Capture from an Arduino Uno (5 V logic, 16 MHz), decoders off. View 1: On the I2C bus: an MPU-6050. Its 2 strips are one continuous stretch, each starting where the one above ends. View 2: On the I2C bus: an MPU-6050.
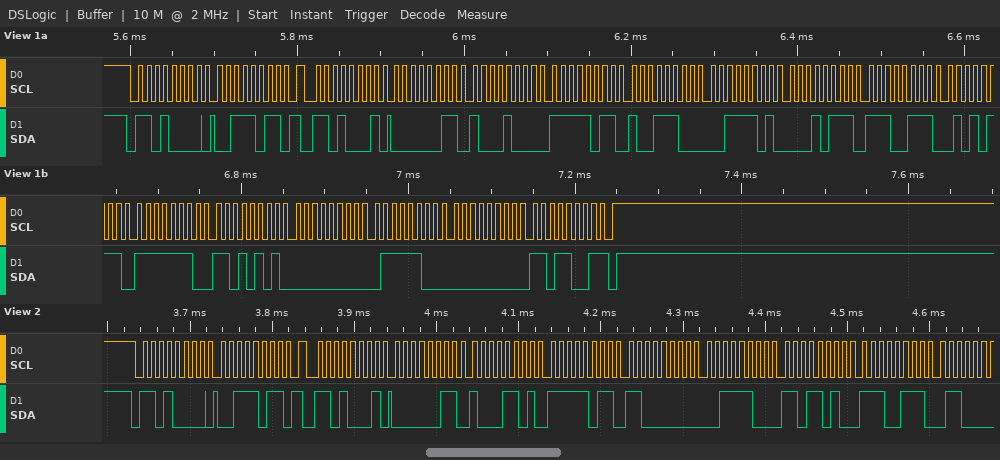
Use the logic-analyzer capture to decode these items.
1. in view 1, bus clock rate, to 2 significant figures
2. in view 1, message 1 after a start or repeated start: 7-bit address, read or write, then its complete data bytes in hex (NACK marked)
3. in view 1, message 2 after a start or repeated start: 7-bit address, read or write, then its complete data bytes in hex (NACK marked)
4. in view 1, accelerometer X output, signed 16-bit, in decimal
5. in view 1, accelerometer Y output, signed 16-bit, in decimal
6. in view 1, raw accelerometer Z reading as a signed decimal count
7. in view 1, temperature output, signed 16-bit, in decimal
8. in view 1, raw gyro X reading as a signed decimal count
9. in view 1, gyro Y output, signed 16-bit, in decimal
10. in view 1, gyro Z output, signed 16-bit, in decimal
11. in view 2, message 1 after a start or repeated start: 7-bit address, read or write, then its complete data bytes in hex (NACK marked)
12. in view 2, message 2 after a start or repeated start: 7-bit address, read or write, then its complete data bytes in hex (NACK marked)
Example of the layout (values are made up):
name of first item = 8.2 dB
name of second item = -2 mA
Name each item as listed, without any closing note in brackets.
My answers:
in view 1, bus clock rate, to 2 significant figures = 100 kHz
in view 1, message 1 after a start or repeated start: 7-bit address, read or write, then its complete data bytes in hex = 0x68 write: 3B
in view 1, message 2 after a start or repeated start: 7-bit address, read or write, then its complete data bytes in hex = 0x68 read: 03 88 FB 9C 3D 17 E7 57 FE D5 00 7C 00 D9 NACK
in view 1, accelerometer X output, signed 16-bit, in decimal = 904
in view 1, accelerometer Y output, signed 16-bit, in decimal = -1124
in view 1, raw accelerometer Z reading as a signed decimal count = 15639
in view 1, temperature output, signed 16-bit, in decimal = -6313
in view 1, raw gyro X reading as a signed decimal count = -299
in view 1, gyro Y output, signed 16-bit, in decimal = 124
in view 1, gyro Z output, signed 16-bit, in decimal = 217
in view 2, message 1 after a start or repeated start: 7-bit address, read or write, then its complete data bytes in hex = 0x68 write: 3B
in view 2, message 2 after a start or repeated start: 7-bit address, read or write, then its complete data bytes in hex = 0x68 read: 03 8D FB C0 3C DA E7
